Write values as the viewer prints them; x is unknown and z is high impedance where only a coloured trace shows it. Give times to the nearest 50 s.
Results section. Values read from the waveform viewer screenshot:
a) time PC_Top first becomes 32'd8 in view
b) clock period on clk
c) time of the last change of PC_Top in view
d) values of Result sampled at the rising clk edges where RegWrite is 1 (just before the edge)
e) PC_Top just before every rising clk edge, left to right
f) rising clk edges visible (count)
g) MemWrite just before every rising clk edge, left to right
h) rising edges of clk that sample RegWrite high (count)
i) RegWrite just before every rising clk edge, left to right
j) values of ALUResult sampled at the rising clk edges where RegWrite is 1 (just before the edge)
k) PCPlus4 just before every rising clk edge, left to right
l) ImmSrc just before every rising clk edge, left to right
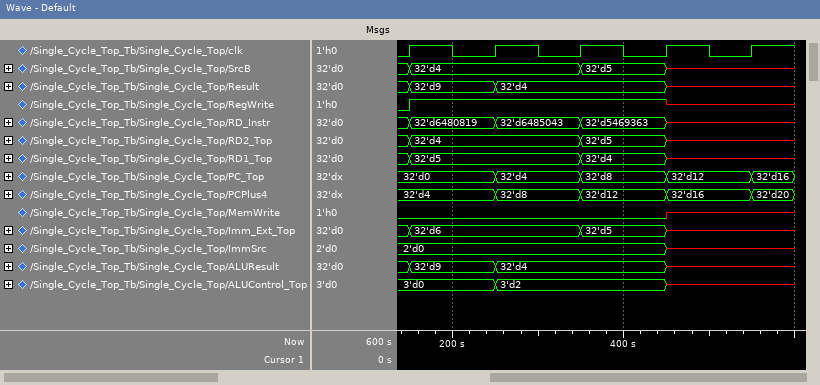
350 s
100 s
550 s
32'd9, 32'd4, 32'd4
32'd0, 32'd0, 32'd4, 32'd8, 32'd12
5
0 0 0 0 x
3
0 1 1 1 x
32'd9, 32'd4, 32'd4
32'd4, 32'd4, 32'd8, 32'd12, 32'd16
2'd0, 2'd0, 2'd0, 2'd0, x
